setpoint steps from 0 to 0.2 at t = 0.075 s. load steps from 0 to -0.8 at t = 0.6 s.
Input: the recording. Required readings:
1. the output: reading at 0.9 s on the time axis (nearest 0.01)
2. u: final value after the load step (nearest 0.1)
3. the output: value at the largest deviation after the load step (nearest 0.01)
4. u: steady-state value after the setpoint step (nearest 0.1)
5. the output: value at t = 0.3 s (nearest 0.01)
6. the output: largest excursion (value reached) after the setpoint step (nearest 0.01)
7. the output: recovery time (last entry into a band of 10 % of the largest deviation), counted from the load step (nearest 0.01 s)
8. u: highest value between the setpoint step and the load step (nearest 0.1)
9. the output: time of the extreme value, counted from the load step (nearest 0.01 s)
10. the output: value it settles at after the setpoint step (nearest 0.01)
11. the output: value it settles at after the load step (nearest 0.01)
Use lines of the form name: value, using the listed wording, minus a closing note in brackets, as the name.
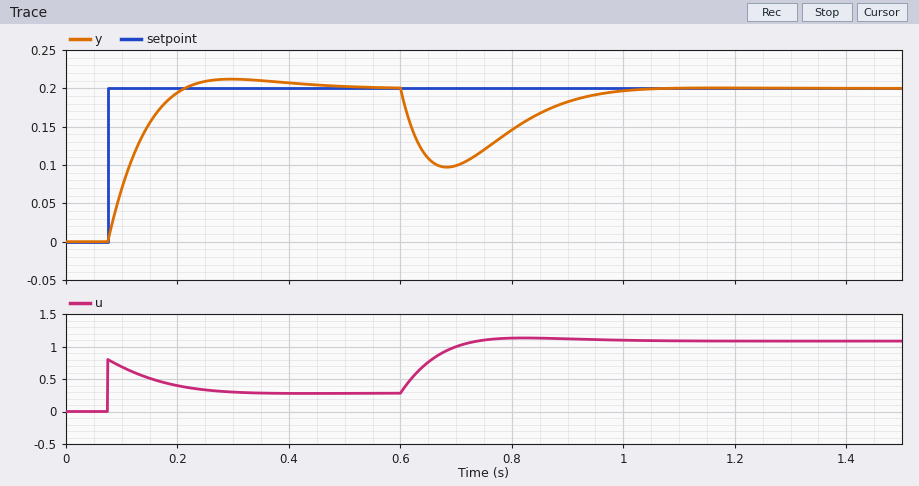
the output: reading at 0.9 s on the time axis: 0.18
u: final value after the load step: 1.1
the output: value at the largest deviation after the load step: 0.10
u: steady-state value after the setpoint step: 0.3
the output: value at t = 0.3 s: 0.21
the output: largest excursion (value reached) after the setpoint step: 0.21
the output: recovery time (last entry into a band of 10 % of the largest deviation), counted from the load step: 0.34 s
u: highest value between the setpoint step and the load step: 0.8
the output: time of the extreme value, counted from the load step: 0.08 s
the output: value it settles at after the setpoint step: 0.20
the output: value it settles at after the load step: 0.20
